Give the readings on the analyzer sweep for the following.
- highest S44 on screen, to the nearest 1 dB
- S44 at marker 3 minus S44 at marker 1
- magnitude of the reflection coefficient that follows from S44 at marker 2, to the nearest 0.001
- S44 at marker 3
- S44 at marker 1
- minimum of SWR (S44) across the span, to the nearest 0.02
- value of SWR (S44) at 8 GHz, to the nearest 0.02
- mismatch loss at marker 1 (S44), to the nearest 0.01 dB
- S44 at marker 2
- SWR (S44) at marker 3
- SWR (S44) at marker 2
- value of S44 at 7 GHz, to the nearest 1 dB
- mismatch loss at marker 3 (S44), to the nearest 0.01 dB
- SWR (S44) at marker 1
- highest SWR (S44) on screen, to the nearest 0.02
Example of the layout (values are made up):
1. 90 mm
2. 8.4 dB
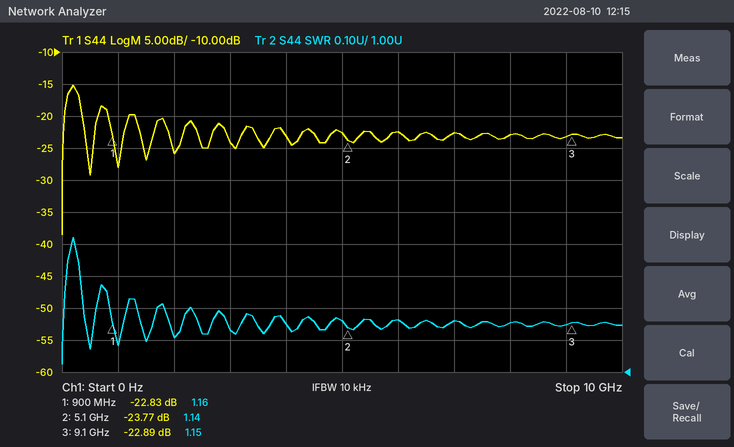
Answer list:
1. -15 dB
2. -0.06 dB
3. 0.065
4. -22.89 dB
5. -22.83 dB
6. 1.02
7. 1.16
8. 0.02 dB
9. -23.77 dB
10. 1.15
11. 1.14
12. -23 dB
13. 0.02 dB
14. 1.16
15. 1.42
